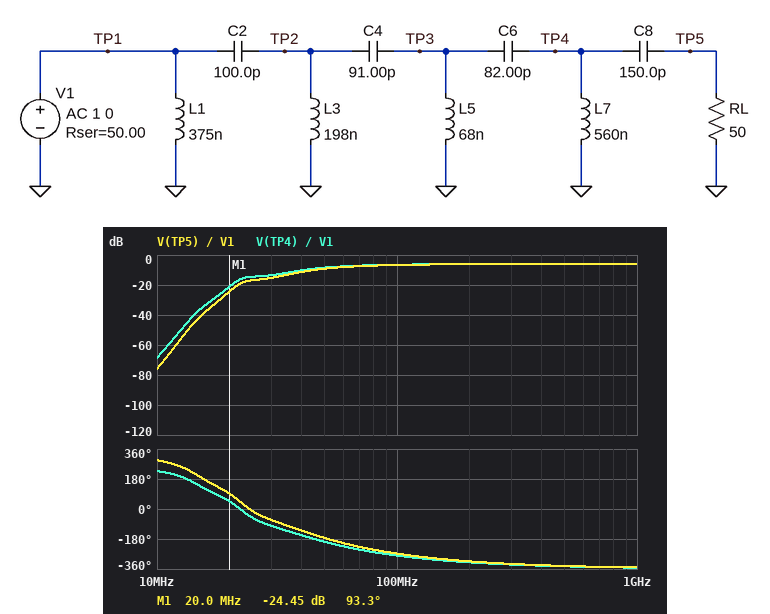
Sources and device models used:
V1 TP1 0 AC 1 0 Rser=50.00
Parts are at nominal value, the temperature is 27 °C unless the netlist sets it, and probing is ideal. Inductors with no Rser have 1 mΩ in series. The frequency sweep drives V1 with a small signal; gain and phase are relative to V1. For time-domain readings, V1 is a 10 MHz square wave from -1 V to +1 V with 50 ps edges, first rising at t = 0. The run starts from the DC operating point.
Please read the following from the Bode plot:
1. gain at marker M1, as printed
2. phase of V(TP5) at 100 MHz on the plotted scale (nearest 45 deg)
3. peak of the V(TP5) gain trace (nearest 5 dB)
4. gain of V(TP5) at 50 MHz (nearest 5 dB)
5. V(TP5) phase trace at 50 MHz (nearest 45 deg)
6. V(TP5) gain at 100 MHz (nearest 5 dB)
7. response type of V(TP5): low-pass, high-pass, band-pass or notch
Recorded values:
-24.45 dB
-270 deg
-5 dB
-10 dB
-180 deg
-5 dB
high-pass
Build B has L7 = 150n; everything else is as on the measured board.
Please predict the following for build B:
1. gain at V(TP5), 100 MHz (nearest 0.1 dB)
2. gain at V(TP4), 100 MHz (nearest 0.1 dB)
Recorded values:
-6.8 dB
-6.6 dB
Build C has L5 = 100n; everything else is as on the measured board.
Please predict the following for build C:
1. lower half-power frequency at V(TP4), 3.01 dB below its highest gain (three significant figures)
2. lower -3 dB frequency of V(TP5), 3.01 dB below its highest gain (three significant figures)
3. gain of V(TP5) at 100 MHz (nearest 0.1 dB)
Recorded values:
32.7 MHz
37.5 MHz
-6.2 dB
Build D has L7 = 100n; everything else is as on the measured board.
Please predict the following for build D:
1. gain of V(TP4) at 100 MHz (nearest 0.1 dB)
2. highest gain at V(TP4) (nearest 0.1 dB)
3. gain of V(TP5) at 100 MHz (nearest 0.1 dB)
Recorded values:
-6.8 dB
-5.4 dB
-7.0 dB
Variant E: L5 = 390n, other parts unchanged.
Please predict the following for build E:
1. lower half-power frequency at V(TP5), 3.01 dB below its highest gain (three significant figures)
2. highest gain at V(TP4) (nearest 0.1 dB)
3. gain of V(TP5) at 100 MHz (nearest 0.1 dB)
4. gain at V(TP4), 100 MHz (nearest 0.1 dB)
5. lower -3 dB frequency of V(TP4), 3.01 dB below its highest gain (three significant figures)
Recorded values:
18.4 MHz
-3.7 dB
-6.2 dB
-6.0 dB
17.8 MHz
